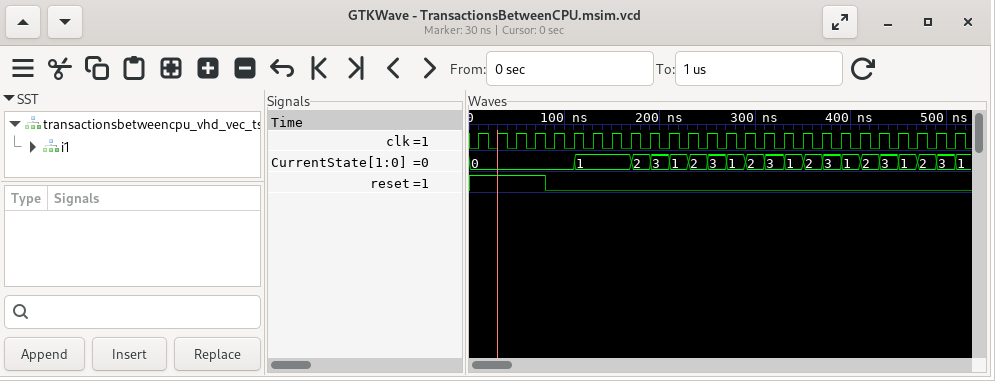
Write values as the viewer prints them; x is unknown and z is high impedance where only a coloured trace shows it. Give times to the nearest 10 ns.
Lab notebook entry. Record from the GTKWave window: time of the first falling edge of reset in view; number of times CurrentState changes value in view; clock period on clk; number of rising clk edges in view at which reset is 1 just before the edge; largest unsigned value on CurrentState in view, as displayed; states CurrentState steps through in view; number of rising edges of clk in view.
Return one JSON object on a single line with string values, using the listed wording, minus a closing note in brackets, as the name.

{"time of the first falling edge of reset in view": "80 ns", "number of times CurrentState changes value in view": "19", "clock period on clk": "20 ns", "number of rising clk edges in view at which reset is 1 just before the edge": "4", "largest unsigned value on CurrentState in view, as displayed": "3", "states CurrentState steps through in view": "0, 1, 2, 3, 1, 2, 3, 1, 2, 3, 1, 2, 3, 1, 2, 3, 1, 2, 3, 1", "number of rising edges of clk in view": "26"}
